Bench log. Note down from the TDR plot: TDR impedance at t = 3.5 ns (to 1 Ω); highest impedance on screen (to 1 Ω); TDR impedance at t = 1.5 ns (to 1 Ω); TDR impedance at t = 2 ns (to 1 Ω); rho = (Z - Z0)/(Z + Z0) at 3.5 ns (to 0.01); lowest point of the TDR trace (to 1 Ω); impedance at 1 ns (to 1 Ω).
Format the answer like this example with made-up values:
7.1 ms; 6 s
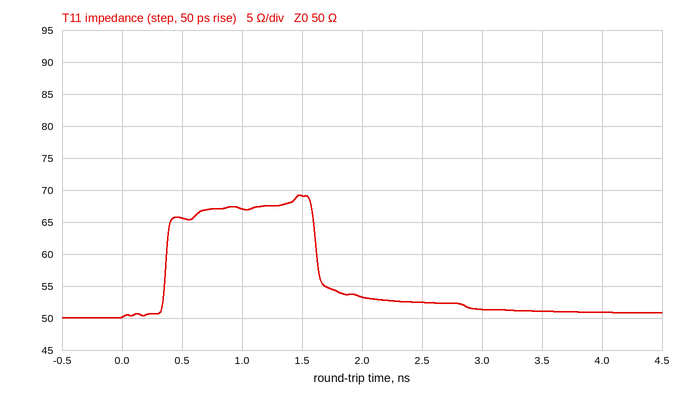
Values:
51 Ω; 69 Ω; 69 Ω; 53 Ω; +0.01; 50 Ω; 67 Ω
